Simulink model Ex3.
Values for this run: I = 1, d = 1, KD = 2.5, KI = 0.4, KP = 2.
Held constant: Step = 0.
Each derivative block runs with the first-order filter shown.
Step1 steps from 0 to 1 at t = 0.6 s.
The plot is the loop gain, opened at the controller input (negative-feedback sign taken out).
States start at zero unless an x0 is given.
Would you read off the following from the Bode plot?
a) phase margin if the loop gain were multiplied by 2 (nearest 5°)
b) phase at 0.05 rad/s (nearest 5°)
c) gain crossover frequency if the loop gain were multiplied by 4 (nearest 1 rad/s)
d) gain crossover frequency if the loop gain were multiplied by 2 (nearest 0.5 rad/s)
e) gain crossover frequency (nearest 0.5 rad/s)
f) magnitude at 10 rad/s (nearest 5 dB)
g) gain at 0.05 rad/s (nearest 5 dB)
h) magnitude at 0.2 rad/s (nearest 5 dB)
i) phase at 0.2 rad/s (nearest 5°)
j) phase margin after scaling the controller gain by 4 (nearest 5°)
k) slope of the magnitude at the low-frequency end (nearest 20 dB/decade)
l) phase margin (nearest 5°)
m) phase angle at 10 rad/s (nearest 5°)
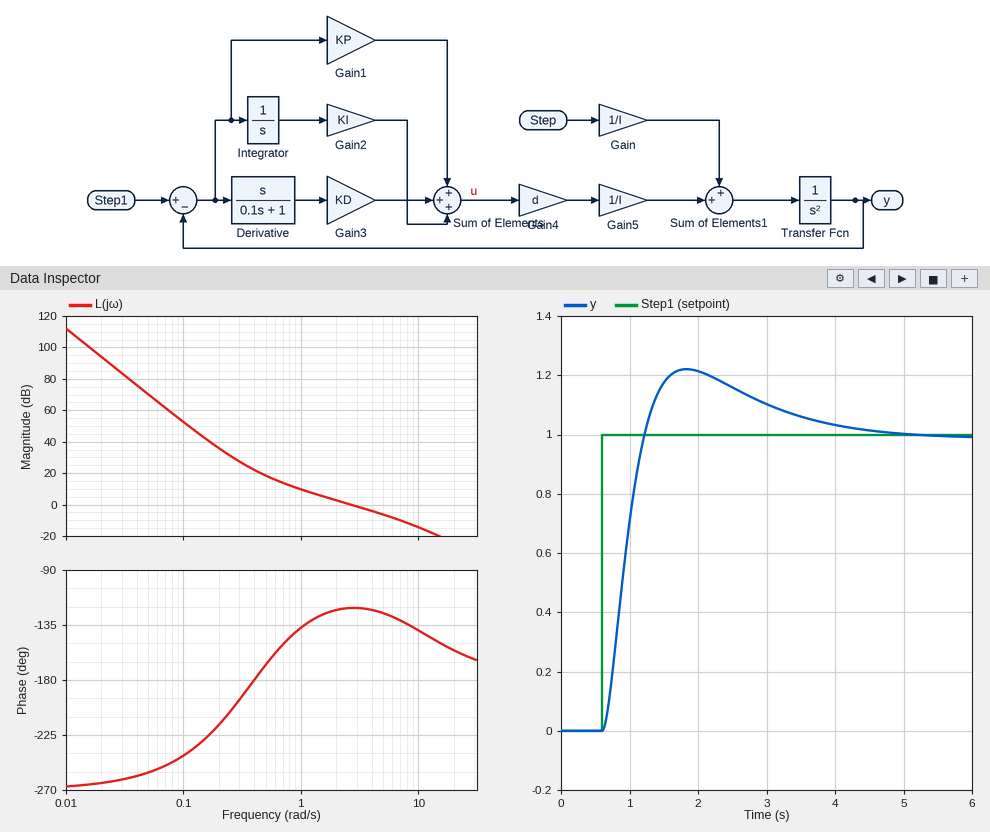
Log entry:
55°
-255°
8 rad/s
5.0 rad/s
2.5 rad/s
-15 dB
70 dB
35 dB
-215°
45°
-60 dB/decade
60°
-140°
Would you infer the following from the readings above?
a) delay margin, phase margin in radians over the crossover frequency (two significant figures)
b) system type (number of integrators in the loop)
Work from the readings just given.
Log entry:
0.42 s
3
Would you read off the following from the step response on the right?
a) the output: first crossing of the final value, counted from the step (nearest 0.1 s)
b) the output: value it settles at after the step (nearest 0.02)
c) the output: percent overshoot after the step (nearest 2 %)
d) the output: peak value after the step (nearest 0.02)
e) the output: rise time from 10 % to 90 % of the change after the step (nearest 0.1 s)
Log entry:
0.6 s
1.00
22 %
1.22
0.4 s
